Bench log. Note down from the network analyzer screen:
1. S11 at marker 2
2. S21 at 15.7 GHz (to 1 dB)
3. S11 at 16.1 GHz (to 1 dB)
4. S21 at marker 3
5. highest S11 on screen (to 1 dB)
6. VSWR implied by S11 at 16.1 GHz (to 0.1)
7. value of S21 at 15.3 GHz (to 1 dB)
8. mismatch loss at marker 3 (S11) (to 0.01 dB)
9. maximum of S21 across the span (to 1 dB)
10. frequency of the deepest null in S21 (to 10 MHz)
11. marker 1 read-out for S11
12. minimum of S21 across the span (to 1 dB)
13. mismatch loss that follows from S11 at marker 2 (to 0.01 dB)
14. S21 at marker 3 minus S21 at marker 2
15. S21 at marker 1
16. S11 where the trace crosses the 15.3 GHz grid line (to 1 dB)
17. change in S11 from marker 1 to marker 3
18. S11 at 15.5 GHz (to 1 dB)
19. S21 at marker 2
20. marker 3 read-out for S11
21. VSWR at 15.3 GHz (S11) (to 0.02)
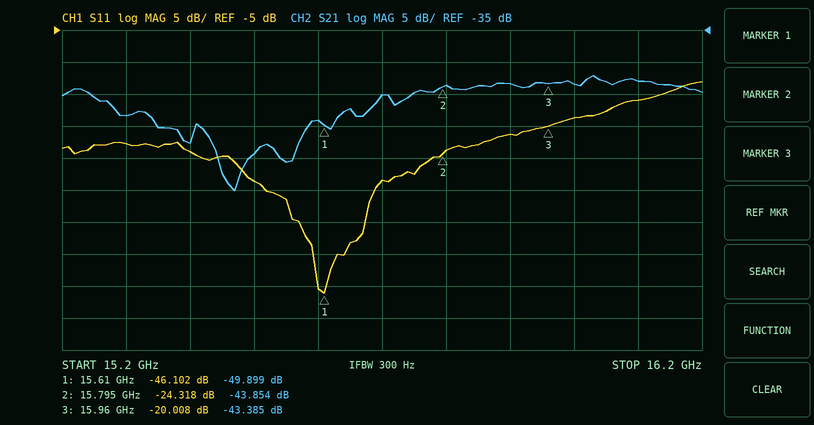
-24.318 dB
-45 dB
-16 dB
-43.385 dB
-13 dB
1.4
-48 dB
0.04 dB
-42 dB
15.47 GHz
-46.102 dB
-60 dB
0.02 dB
0.469 dB
-49.899 dB
-23 dB
26.094 dB
-29 dB
-43.854 dB
-20.008 dB
1.16
